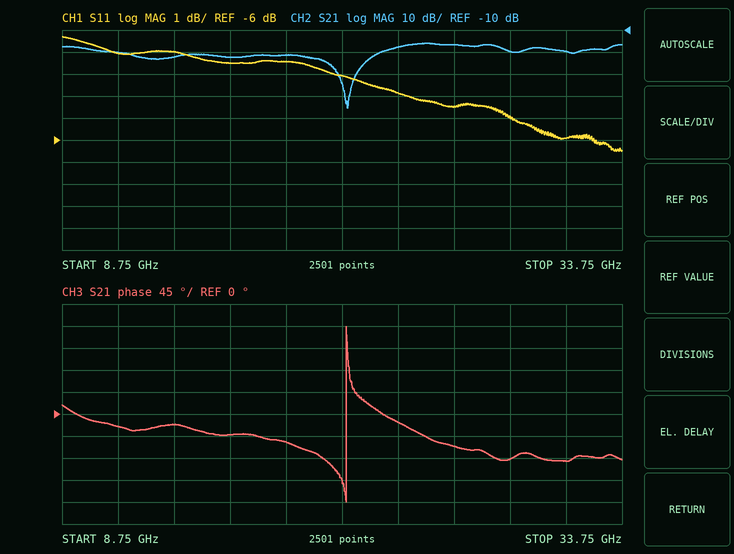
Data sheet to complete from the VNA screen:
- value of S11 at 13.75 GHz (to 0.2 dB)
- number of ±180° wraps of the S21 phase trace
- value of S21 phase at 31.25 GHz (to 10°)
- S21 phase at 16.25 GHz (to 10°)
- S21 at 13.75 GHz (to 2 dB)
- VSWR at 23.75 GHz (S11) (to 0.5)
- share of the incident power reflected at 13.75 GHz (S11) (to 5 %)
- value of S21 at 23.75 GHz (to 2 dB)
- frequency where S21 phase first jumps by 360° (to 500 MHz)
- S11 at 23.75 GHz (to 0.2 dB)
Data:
-2.0 dB
1
-100°
-40°
-22 dB
4.5
65 %
-18 dB
21.5 GHz
-3.8 dB
